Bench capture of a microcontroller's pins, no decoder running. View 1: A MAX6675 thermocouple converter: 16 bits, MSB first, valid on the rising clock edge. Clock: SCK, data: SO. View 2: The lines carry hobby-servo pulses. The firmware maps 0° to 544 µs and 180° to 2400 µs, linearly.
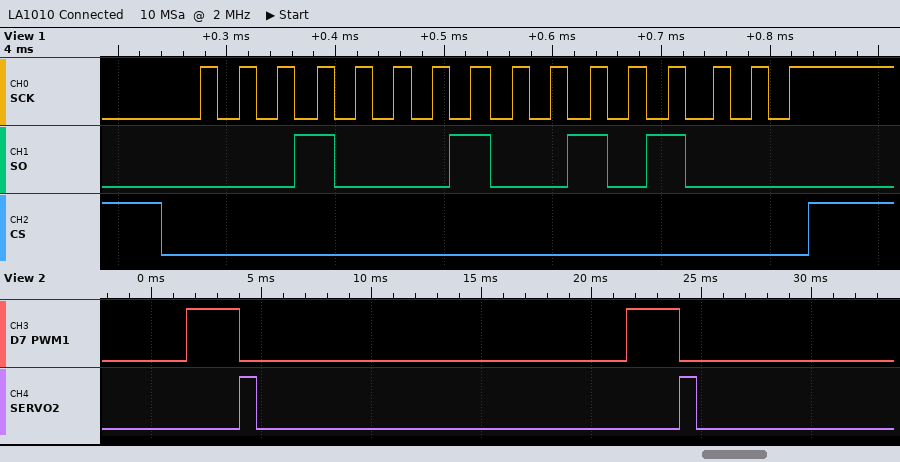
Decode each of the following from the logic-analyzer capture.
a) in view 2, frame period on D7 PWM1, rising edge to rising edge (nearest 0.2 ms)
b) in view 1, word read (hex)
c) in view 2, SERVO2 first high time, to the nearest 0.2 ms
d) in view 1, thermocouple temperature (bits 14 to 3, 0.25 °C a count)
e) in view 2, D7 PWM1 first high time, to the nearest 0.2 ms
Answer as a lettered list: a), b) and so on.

a) 20.0 ms
b) 0x1128
c) 0.8 ms
d) 137.25 °C
e) 2.4 ms
